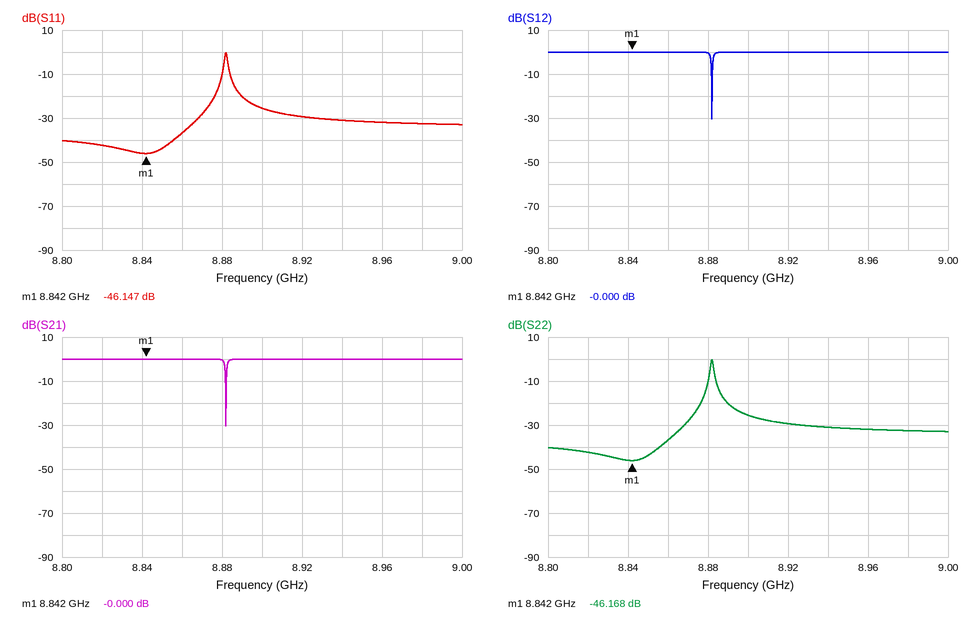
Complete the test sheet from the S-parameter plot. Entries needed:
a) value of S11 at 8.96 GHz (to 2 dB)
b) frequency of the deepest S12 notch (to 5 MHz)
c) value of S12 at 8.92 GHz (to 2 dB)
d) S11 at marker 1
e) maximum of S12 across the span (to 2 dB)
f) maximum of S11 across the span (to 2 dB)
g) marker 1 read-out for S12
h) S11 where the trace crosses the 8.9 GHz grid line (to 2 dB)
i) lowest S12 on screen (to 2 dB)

-32 dB
8.880 GHz
0 dB
-46.147 dB
0 dB
0 dB
-0.000 dB
-26 dB
-30 dB
